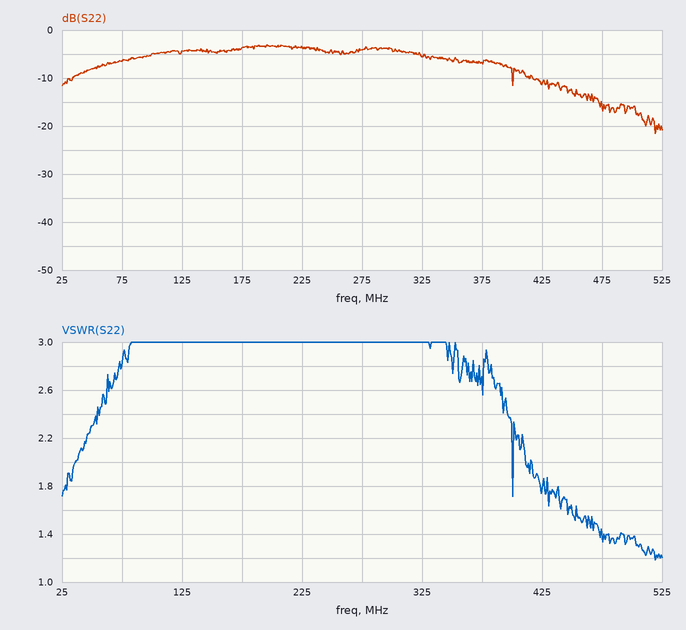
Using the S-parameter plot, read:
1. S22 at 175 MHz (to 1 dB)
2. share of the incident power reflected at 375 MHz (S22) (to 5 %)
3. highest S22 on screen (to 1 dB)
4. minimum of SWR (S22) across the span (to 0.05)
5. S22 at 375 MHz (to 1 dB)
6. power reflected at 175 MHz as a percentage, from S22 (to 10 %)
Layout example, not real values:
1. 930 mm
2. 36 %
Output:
1. -4 dB
2. 20 %
3. -3 dB
4. 1.20
5. -7 dB
6. 40 %
